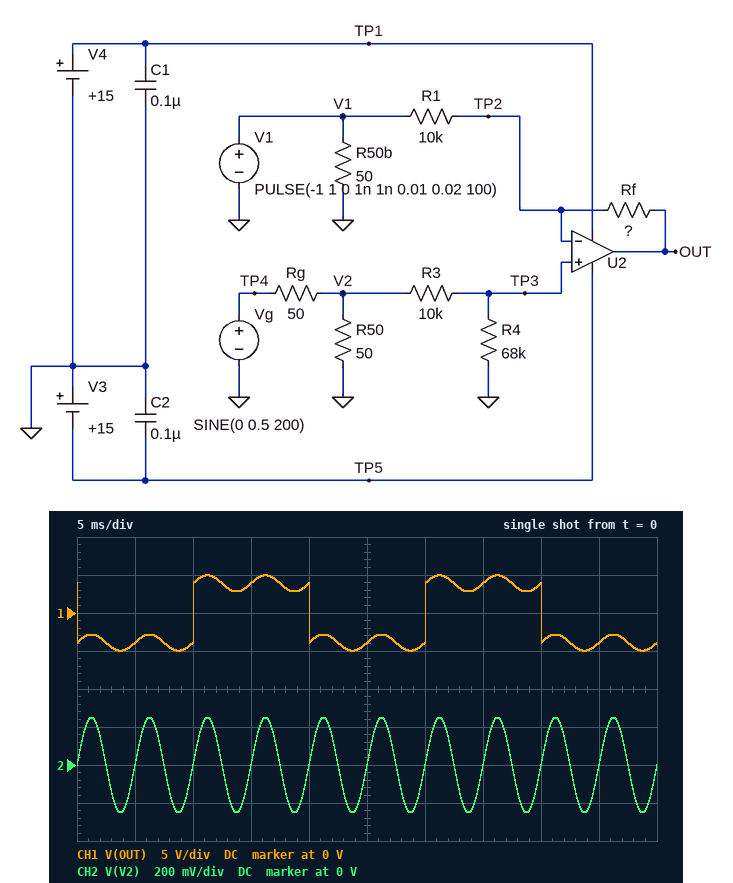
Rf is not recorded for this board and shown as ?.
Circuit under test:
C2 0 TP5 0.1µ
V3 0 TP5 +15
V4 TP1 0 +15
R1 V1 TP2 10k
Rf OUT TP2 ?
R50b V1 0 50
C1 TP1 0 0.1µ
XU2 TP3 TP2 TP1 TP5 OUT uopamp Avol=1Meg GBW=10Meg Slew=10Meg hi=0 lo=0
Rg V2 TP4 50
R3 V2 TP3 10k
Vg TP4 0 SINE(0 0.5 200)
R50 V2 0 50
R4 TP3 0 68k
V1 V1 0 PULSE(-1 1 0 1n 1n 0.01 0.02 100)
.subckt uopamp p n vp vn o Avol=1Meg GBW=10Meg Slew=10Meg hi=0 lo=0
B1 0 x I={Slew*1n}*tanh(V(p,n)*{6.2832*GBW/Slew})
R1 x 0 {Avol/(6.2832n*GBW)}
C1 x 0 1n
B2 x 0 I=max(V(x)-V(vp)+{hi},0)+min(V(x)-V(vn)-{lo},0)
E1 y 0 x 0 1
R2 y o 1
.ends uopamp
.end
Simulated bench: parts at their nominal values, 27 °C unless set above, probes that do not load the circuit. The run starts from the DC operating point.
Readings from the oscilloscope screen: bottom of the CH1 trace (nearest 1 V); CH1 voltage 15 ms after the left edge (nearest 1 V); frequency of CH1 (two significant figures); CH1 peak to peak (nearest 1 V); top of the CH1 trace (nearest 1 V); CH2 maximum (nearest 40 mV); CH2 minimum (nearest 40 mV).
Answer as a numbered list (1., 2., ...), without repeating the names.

1. -5 V
2. 4 V
3. 50 Hz
4. 10 V
5. 5 V
6. 240 mV
7. -240 mV
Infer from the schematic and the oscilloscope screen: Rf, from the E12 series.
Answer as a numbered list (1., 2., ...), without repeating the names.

1. 39 kΩ
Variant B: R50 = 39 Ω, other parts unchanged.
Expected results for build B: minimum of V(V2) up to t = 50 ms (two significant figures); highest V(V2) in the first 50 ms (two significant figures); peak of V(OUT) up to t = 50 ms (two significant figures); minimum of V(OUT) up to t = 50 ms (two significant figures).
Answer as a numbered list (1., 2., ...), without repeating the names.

1. -220 mV
2. 220 mV
3. 4.8 V
4. -4.8 V
